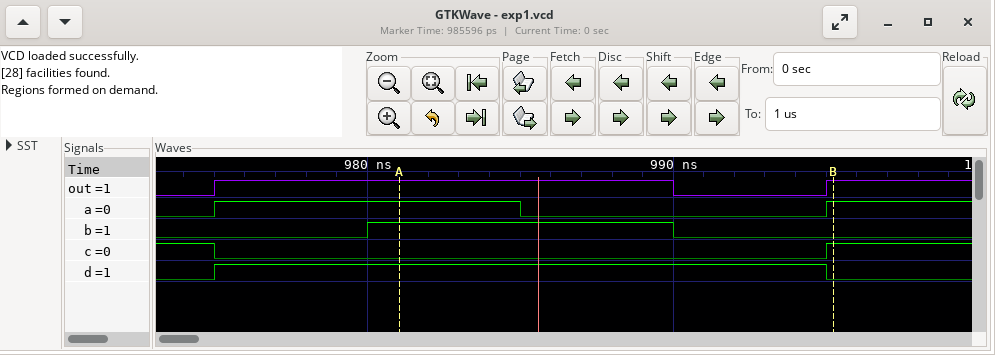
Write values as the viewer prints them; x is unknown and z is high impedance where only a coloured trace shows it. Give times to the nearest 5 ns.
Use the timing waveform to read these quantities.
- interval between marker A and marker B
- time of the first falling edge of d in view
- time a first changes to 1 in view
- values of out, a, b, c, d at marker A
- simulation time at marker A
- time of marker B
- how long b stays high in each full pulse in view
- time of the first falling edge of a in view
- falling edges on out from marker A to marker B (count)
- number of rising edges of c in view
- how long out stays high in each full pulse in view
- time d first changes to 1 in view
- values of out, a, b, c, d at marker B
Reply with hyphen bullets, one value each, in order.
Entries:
- 15 ns
- 995 ns
- 975 ns
- out=1, a=1, b=1, c=0, d=1
- 980 ns
- 995 ns
- 10 ns
- 985 ns
- 1
- 1
- 15 ns
- 975 ns
- out=1, a=1, b=0, c=1, d=0
